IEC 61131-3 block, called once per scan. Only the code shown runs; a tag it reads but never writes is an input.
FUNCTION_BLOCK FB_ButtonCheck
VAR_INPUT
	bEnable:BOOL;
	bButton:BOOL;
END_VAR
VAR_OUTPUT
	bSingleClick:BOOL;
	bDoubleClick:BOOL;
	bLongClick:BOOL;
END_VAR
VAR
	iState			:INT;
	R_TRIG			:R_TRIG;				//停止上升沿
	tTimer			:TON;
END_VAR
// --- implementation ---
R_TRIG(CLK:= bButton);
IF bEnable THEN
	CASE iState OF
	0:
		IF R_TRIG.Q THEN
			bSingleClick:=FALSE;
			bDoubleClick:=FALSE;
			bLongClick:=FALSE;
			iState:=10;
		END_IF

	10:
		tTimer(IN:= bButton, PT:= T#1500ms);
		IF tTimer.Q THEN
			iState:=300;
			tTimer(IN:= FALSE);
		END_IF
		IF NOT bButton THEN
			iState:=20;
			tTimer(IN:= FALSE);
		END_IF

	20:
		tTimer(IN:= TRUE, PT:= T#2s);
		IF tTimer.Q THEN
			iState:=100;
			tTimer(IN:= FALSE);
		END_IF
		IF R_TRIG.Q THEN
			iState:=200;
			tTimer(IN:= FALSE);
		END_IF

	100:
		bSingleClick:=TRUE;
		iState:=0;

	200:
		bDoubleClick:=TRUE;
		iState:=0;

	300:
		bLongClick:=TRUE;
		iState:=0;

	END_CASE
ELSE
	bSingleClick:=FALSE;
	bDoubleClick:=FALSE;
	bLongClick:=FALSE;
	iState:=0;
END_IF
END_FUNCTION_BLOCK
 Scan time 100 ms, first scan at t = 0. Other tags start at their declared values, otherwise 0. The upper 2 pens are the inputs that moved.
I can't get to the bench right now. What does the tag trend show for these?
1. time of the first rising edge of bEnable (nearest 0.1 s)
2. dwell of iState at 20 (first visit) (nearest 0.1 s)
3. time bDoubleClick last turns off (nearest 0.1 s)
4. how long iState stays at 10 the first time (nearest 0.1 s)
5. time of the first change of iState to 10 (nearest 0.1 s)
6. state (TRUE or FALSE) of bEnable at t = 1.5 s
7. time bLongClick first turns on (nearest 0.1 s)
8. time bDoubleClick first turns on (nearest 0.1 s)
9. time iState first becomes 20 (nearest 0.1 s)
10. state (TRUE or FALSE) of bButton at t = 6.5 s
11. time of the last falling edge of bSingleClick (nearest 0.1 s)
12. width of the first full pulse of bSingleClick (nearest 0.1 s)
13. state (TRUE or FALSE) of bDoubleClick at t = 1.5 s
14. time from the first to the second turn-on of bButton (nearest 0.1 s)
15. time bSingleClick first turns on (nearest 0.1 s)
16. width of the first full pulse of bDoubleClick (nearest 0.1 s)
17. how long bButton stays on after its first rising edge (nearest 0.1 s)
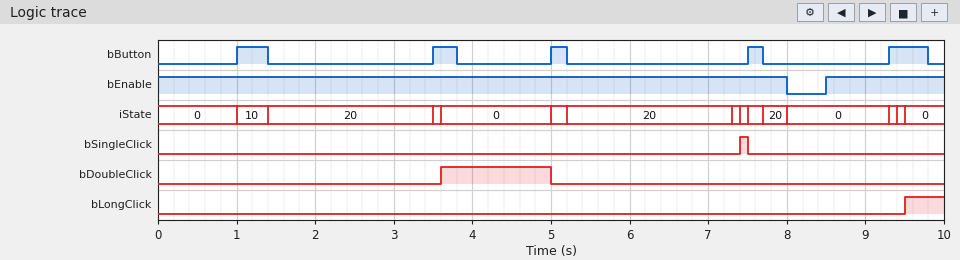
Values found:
8.5 s
2.1 s
5.0 s
0.4 s
1.0 s
TRUE
9.5 s
3.6 s
1.4 s
FALSE
7.5 s
0.1 s
FALSE
2.5 s
7.4 s
1.4 s
0.4 s
